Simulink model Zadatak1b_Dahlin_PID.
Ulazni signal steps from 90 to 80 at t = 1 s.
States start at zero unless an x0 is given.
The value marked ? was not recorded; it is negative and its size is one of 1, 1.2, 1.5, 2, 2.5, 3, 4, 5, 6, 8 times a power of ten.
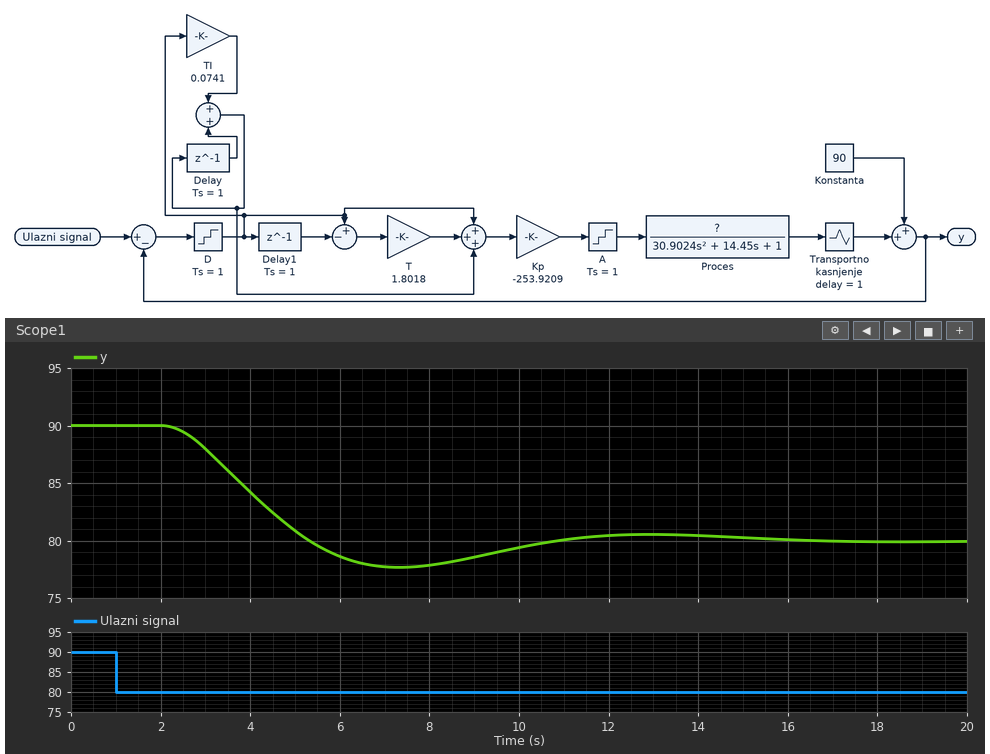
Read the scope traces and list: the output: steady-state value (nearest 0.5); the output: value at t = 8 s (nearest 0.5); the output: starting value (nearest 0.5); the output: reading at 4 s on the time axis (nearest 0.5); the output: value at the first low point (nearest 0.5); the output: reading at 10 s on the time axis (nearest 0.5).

80.0
78.0
90.0
84.0
77.5
79.5
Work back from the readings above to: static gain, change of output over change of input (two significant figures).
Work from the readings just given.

1.0
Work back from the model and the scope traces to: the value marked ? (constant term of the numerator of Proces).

-0.02
